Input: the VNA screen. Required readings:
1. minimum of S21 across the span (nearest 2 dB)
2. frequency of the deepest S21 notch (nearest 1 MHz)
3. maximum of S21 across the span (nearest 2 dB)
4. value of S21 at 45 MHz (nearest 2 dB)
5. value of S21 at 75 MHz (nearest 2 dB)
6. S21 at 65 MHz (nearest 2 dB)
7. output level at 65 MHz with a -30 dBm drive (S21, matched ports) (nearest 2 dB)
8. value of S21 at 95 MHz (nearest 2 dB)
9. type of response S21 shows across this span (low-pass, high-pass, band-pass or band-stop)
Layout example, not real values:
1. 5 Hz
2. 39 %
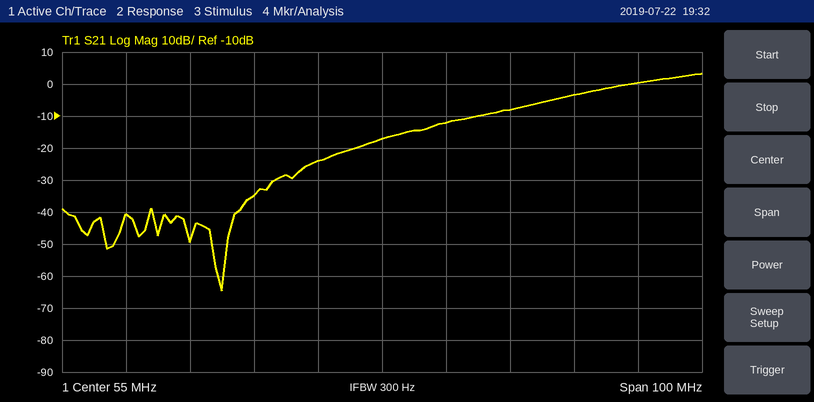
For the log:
1. -64 dB
2. 30 MHz
3. 4 dB
4. -24 dB
5. -8 dB
6. -12 dB
7. -42 dBm
8. 0 dB
9. high-pass
